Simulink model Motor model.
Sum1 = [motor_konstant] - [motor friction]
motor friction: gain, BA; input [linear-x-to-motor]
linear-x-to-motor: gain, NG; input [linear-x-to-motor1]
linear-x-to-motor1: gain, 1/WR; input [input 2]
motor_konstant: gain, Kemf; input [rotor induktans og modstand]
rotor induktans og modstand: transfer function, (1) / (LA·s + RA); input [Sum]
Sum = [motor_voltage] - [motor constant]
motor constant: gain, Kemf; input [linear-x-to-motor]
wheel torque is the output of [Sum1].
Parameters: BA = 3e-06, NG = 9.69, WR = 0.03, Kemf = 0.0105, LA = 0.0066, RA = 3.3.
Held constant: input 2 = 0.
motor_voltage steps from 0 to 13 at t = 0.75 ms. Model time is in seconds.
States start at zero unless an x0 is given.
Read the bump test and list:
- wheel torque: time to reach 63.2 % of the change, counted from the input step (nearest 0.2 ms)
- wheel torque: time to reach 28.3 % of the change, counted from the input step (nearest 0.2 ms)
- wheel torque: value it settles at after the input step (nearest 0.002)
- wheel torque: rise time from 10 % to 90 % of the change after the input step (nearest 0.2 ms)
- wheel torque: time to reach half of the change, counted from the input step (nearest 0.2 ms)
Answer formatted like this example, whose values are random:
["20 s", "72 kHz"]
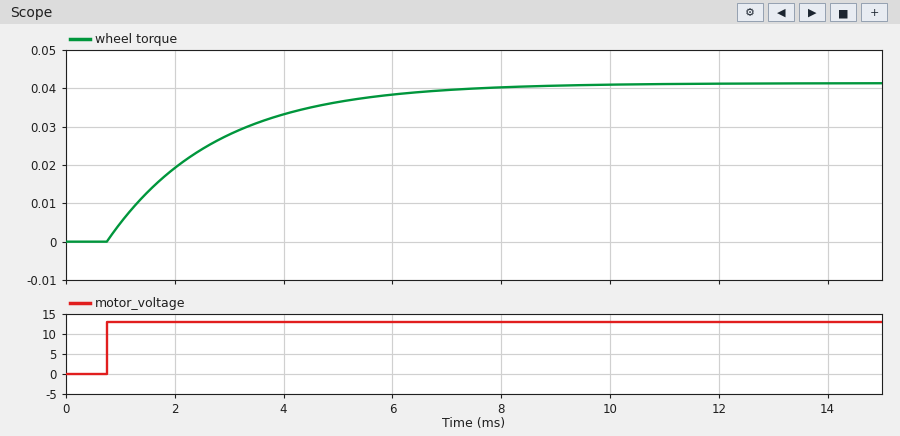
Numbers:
["2.0 ms", "0.6 ms", "0.042", "4.4 ms", "1.4 ms"]
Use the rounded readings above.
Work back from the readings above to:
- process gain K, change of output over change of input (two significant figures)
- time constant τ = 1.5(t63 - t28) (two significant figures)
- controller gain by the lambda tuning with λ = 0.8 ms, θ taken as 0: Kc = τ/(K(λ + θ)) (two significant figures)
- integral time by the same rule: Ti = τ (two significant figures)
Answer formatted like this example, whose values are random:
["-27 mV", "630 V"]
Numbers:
["0.0032", "2.1 ms", "820", "2.1 ms"]
